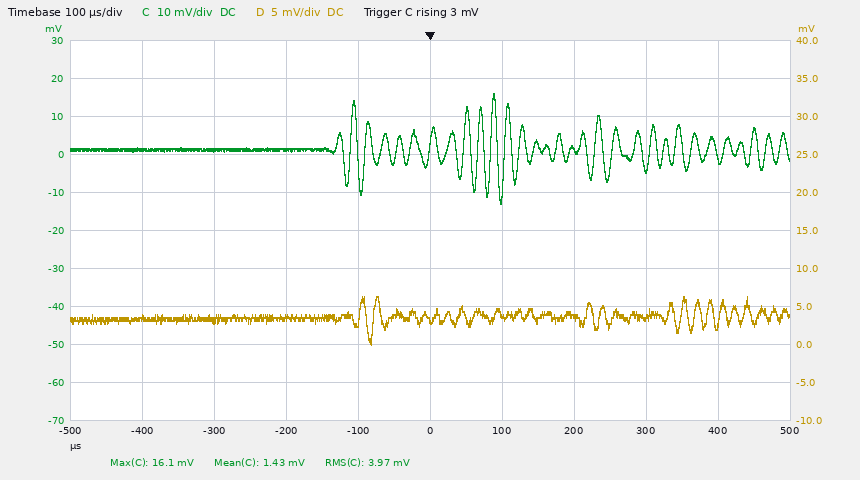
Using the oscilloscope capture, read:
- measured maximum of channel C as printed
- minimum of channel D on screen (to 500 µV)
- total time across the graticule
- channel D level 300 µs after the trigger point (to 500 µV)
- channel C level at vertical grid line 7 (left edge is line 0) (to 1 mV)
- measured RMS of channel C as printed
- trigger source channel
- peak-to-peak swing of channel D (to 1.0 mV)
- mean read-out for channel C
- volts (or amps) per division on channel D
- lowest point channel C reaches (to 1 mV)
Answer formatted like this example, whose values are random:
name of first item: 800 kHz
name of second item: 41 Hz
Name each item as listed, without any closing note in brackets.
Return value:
measured maximum of channel C as printed: 16.1 mV
minimum of channel D on screen: 0.0 mV
total time across the graticule: 1 ms
channel D level 300 µs after the trigger point: 3.5 mV
channel C level at vertical grid line 7 (left edge is line 0): 1 mV
measured RMS of channel C as printed: 3.97 mV
trigger source channel: channel C
peak-to-peak swing of channel D: 6.0 mV
mean read-out for channel C: 1.43 mV
volts (or amps) per division on channel D: 5 mV
lowest point channel C reaches: -13 mV
